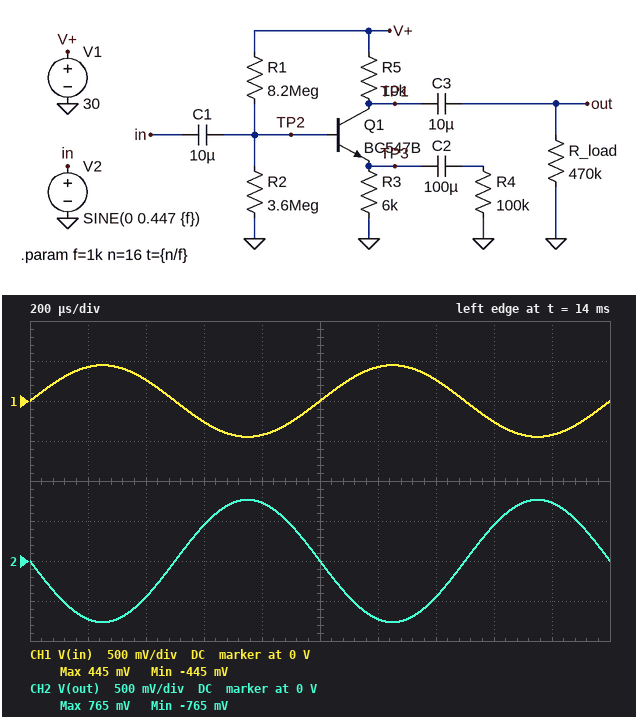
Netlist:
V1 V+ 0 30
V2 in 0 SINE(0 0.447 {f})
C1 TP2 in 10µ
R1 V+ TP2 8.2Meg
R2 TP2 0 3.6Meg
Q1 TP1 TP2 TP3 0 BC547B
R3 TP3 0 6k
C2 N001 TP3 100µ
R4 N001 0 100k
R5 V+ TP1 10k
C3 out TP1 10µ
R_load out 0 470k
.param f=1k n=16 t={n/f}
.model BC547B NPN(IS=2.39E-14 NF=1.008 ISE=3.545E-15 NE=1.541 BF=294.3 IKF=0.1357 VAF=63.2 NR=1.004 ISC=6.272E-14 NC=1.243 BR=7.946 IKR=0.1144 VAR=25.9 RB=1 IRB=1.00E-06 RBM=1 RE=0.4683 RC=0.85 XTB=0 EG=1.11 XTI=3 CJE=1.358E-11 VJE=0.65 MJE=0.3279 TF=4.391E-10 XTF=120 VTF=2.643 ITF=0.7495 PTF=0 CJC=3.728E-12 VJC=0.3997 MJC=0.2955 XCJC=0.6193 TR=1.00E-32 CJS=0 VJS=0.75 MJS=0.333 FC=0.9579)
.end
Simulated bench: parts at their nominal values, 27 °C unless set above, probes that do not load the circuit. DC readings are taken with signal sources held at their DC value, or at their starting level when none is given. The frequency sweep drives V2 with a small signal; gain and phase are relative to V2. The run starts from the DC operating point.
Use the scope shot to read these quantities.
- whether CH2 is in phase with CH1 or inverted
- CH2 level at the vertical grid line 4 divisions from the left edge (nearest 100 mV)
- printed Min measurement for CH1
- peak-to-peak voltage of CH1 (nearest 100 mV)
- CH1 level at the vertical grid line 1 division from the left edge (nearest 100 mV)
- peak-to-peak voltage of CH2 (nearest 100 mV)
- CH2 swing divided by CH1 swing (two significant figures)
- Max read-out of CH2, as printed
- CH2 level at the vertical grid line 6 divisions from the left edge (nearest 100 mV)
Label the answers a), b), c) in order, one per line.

a) inverted
b) 700 mV
c) -445 mV
d) 900 mV
e) 400 mV
f) 1.5 V
g) 1.7
h) 765 mV
i) -700 mV
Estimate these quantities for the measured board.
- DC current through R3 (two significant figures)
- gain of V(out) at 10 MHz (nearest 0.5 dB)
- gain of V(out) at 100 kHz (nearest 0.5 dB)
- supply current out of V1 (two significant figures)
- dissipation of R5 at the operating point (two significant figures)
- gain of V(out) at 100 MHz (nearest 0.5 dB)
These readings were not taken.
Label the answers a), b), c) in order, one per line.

a) 670 µA
b) 4.0 dB
c) 4.5 dB
d) 670 µA
e) 4.4 mW
f) 1.0 dB
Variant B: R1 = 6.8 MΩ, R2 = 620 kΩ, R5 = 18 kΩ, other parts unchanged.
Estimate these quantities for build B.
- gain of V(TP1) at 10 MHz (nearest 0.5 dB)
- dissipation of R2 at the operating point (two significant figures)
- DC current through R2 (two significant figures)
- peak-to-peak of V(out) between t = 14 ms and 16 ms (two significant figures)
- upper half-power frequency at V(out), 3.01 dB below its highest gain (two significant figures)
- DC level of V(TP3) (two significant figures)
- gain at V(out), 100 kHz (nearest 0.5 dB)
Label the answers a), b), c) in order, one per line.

a) 6.5 dB
b) 7.3 µW
c) 3.4 µA
d) 2.7 V
e) 10 MHz
f) 1.5 V
g) 9.5 dB
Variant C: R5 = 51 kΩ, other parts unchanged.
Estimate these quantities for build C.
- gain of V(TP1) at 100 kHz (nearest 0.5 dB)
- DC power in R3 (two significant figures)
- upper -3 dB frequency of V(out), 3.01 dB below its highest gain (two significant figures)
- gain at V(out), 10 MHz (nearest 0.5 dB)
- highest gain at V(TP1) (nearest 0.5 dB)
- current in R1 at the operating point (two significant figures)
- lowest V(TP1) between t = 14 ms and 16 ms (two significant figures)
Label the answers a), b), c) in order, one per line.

a) 13.5 dB
b) 1.7 mW
c) 230 kHz
d) 0 dB
e) 14.0 dB
f) 3.2 µA
g) 3.3 V
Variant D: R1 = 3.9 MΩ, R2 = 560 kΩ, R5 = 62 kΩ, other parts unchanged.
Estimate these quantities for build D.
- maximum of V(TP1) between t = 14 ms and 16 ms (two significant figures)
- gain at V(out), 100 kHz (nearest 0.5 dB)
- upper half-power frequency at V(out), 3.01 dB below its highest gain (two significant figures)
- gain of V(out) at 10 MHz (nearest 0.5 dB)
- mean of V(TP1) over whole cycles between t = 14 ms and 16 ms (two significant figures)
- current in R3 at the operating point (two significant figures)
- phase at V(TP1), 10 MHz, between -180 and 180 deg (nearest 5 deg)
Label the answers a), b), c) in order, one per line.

a) 9.0 V
b) 19.5 dB
c) 1.3 MHz
d) 4.5 dB
e) 5.3 V
f) 410 µA
g) 50 deg
